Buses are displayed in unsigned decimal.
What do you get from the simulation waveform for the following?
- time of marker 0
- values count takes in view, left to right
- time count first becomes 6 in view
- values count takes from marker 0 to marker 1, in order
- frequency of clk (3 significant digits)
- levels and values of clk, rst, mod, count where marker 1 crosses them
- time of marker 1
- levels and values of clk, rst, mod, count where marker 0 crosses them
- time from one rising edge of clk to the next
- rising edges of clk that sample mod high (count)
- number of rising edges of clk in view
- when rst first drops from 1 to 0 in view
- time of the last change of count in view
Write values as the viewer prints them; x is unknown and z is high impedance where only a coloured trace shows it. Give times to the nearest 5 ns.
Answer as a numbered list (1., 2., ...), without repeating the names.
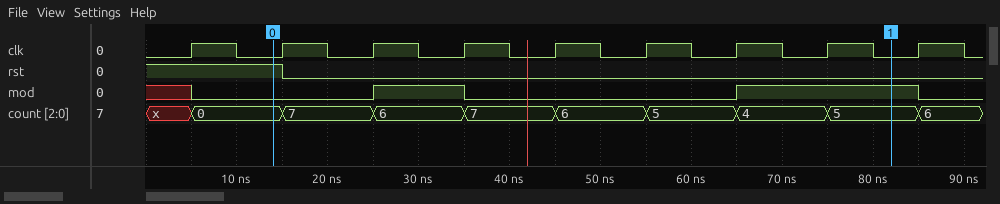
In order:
1. 15 ns
2. x, 0, 7, 6, 7, 6, 5, 4, 5, 6
3. 25 ns
4. 0, 7, 6, 7, 6, 5, 4, 5
5. 100 MHz
6. clk=0, rst=0, mod=1, count=5
7. 80 ns
8. clk=0, rst=1, mod=0, count=0
9. 10 ns
10. 3
11. 9
12. 15 ns
13. 85 ns
